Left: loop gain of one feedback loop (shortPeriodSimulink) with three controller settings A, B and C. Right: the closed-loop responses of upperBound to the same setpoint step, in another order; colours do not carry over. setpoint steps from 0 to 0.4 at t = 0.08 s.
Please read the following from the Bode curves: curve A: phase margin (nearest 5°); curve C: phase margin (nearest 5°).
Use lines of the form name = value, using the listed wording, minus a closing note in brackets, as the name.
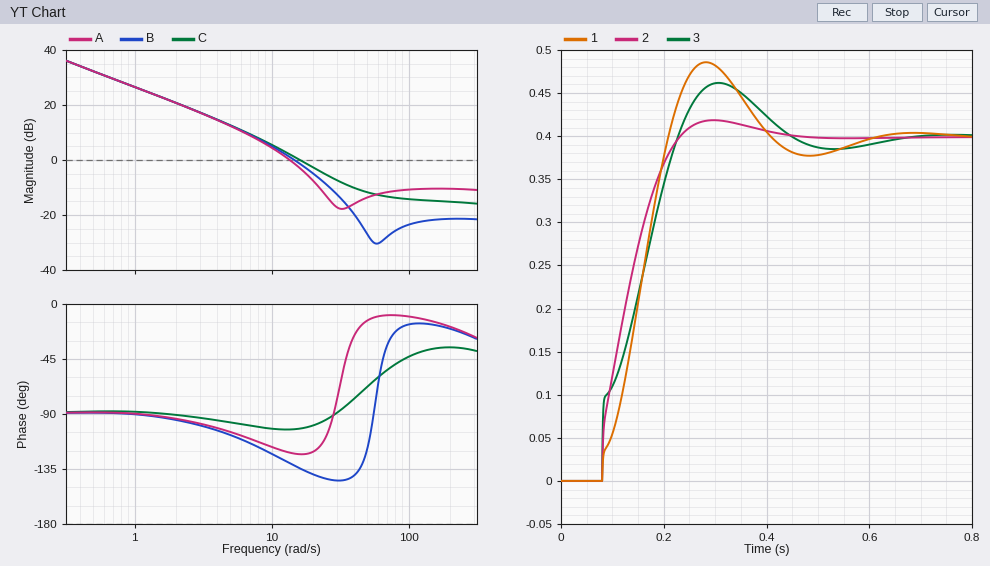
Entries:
curve A: phase margin = 60°
curve C: phase margin = 80°
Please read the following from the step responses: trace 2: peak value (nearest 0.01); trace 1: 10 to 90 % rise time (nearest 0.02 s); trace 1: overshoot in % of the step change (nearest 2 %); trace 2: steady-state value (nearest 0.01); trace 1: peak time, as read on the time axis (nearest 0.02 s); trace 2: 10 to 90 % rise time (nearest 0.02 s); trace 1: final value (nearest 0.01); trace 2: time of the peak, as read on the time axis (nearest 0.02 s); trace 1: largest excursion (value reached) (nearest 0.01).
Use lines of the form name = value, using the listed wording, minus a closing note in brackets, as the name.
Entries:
trace 2: peak value = 0.42
trace 1: 10 to 90 % rise time = 0.10 s
trace 1: overshoot in % of the step change = 22 %
trace 2: steady-state value = 0.40
trace 1: peak time, as read on the time axis = 0.28 s
trace 2: 10 to 90 % rise time = 0.12 s
trace 1: final value = 0.40
trace 2: time of the peak, as read on the time axis = 0.30 s
trace 1: largest excursion (value reached) = 0.49
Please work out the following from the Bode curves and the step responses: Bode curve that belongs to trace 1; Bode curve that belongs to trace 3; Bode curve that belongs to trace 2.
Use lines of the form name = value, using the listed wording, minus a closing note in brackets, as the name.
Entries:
Bode curve that belongs to trace 1 = B
Bode curve that belongs to trace 3 = A
Bode curve that belongs to trace 2 = C
